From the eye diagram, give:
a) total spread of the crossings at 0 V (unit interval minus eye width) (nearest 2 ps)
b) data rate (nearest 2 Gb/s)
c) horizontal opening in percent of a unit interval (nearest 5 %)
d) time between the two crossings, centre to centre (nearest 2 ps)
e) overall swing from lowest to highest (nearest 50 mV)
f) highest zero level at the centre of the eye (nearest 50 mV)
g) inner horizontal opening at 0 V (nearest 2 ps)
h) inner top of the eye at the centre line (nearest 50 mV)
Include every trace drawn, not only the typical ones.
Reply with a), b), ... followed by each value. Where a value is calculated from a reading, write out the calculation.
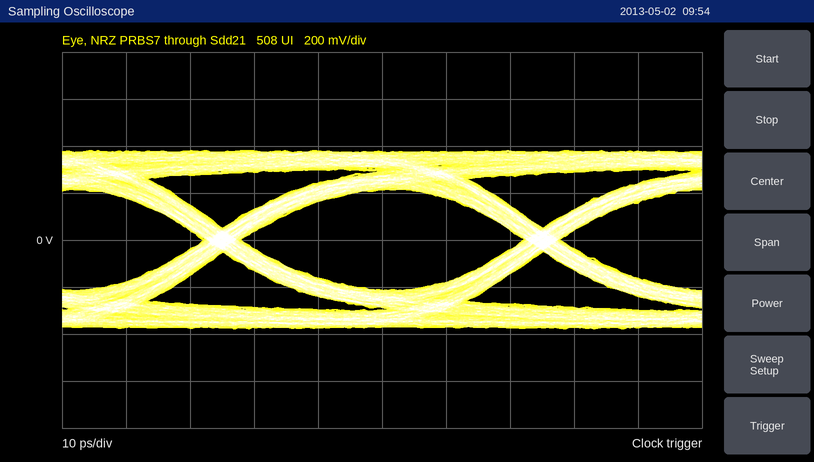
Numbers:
a) 6 ps
b) 20 Gb/s
c) 44 ps / 50 ps ≈ 88.0 %, so 90 % to the nearest 5 %
d) 50 ps
e) 750 mV
f) -200 mV
g) 44 ps
h) 200 mV
